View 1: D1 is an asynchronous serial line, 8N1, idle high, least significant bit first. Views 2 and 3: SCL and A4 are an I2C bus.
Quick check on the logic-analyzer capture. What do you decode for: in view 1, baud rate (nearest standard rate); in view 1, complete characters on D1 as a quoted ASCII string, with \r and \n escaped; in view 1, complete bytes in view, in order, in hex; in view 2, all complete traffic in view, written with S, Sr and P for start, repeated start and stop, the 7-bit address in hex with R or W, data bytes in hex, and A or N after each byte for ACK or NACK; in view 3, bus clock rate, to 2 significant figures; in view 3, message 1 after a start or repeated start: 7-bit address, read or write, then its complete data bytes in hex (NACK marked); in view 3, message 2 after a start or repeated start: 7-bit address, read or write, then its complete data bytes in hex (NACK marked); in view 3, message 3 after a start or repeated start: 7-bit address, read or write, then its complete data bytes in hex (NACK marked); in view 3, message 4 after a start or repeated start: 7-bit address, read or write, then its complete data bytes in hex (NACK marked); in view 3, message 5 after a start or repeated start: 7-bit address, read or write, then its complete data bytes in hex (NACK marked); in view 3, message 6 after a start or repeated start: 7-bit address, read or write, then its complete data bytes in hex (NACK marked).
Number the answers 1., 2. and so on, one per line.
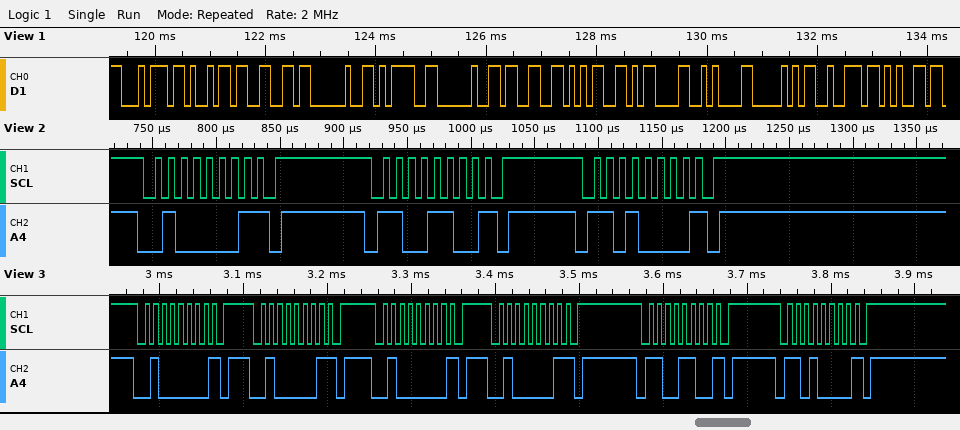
1. 9600 baud
2. "tif = 35\r\nPre"
3. 74 69 66 20 3D 20 33 35 0D 0A 50 72 65
4. S 20R N P S 66W N P S 68W N P
5. 100 kHz
6. 0x20 write NACK
7. 0x20 read NACK
8. 0x20 write NACK
9. 0x20 read NACK
10. 0x66 write NACK
11. 0x68 write NACK
